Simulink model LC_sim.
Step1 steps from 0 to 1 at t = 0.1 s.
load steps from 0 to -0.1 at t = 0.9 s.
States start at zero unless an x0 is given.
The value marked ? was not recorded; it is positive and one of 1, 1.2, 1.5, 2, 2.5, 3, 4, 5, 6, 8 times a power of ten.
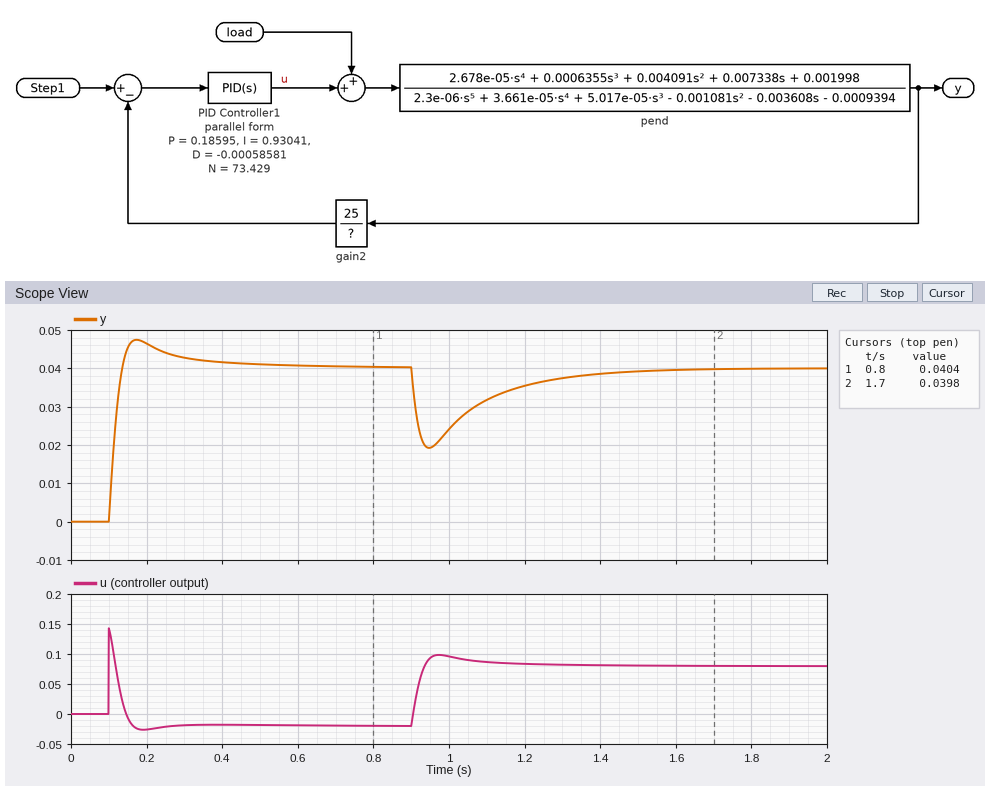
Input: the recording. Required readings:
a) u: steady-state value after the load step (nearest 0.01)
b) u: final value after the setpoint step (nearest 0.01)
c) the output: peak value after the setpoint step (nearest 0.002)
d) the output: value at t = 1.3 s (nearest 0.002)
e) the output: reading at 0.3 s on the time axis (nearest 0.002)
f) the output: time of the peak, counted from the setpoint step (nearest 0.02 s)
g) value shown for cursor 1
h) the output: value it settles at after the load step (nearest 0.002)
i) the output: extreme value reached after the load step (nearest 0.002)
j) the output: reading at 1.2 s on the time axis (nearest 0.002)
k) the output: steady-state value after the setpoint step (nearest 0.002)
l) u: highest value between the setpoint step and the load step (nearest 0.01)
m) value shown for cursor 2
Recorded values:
0.08
-0.02
0.048
0.038
0.042
0.08 s
0.0404
0.040
0.020
0.036
0.040
0.14
0.0398
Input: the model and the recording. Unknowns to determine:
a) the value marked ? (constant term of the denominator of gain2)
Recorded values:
1
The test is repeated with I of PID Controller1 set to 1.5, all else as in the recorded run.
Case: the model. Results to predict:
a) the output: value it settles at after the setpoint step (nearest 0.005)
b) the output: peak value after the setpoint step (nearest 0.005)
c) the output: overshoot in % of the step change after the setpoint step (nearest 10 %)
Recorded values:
0.040
0.050
20 %
